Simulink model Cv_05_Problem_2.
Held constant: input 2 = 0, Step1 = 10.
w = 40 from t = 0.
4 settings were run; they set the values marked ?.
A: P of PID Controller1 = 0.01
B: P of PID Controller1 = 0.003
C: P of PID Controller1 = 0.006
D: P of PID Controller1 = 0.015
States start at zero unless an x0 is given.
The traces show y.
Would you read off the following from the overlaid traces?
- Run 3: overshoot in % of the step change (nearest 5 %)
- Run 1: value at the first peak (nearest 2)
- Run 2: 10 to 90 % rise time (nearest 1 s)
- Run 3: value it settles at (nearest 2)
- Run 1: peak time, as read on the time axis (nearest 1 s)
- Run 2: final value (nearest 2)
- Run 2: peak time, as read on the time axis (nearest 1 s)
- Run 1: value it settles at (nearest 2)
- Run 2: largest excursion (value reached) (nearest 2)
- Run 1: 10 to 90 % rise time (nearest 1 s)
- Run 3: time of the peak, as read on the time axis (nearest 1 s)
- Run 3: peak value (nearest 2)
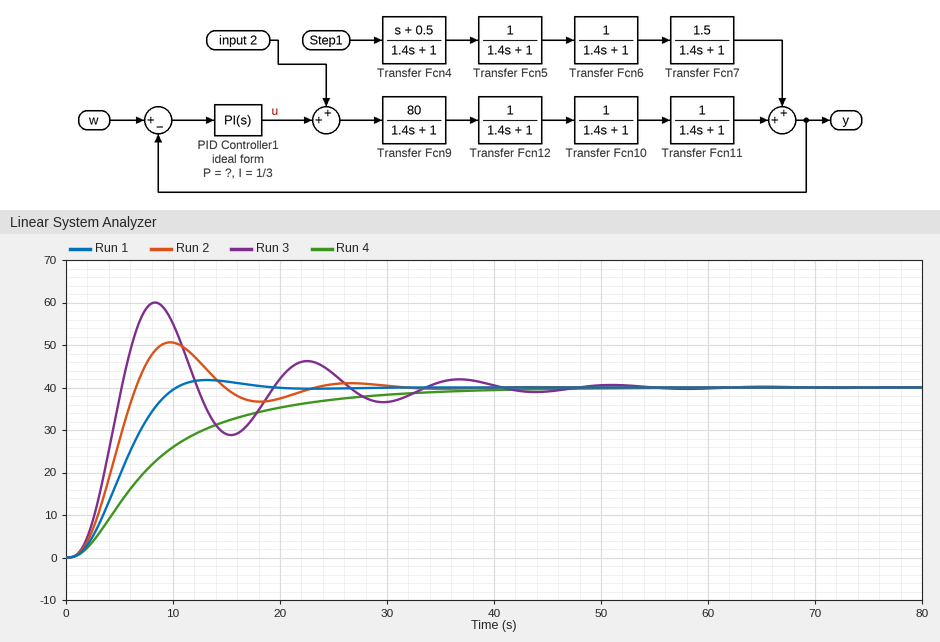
50 %
42
4 s
40
13 s
40
10 s
40
50
6 s
8 s
60
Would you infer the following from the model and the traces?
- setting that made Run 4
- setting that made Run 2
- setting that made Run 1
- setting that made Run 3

B
A
C
D
